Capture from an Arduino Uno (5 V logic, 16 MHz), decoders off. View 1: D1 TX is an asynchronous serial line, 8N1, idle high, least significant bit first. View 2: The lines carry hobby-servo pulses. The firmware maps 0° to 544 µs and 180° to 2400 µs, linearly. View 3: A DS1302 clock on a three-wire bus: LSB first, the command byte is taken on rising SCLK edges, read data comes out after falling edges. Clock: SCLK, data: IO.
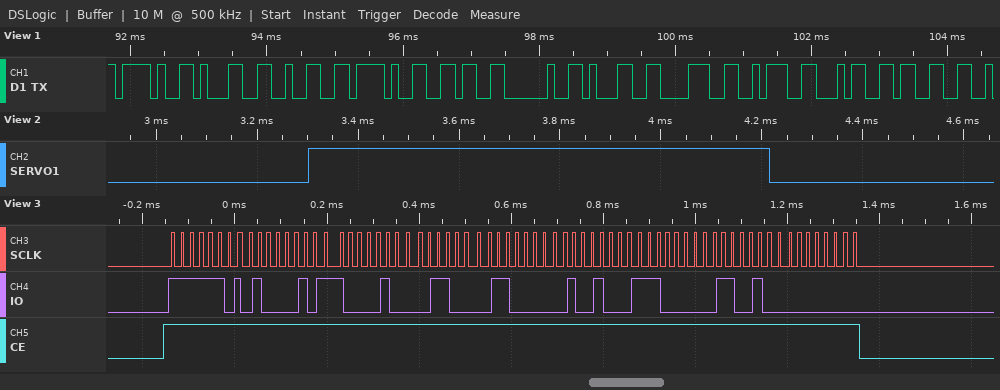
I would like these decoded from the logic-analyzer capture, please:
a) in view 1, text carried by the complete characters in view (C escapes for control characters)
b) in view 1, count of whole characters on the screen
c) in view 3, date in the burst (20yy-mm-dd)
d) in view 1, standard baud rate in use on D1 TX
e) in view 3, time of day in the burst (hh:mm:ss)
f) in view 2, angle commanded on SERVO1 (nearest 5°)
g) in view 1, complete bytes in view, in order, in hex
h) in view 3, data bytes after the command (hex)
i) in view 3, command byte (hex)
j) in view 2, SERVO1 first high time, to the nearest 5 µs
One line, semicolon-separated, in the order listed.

"/12/6 18:43"; 11; 2026-12-06; 9600 baud; 18:43:42; 35°; 2F 31 32 2F 36 20 31 38 3A 34 33; 42 43 18 06 12 07 26 00; 0xBF; 915 µs
